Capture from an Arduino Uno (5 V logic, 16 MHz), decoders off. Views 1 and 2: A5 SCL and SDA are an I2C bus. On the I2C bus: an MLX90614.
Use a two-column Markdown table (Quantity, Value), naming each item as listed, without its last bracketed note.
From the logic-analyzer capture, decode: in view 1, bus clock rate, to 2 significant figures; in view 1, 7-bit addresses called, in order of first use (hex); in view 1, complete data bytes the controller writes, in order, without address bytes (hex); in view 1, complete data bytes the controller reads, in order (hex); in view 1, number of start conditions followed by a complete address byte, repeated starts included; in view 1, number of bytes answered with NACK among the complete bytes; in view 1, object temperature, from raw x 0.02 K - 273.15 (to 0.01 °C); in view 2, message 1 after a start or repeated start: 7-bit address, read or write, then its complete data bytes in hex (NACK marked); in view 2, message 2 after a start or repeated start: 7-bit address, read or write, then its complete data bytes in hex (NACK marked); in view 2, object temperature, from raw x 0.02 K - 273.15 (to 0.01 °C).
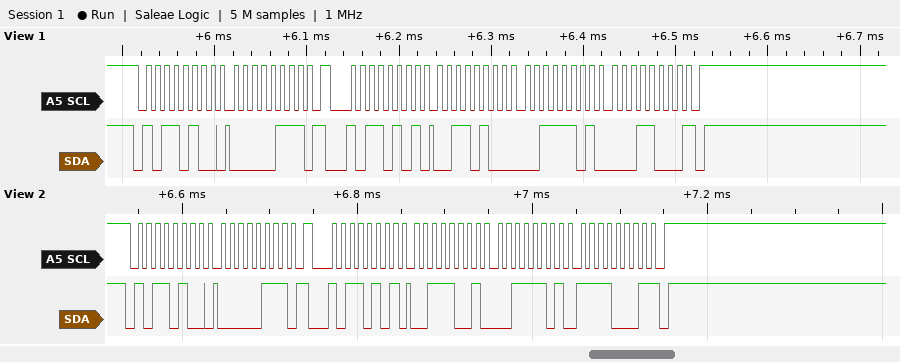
| Quantity | Value |
|---|---|
| in view 1, bus clock rate, to 2 significant figures | 100 kHz |
| in view 1, 7-bit addresses called, in order of first use | 0x5A |
| in view 1, complete data bytes the controller writes, in order, without address bytes | 07 |
| in view 1, complete data bytes the controller reads, in order | 34 3D 18 |
| in view 1, number of start conditions followed by a complete address byte, repeated starts included | 2 |
| in view 1, number of bytes answered with NACK among the complete bytes | 1 |
| in view 1, object temperature, from raw x 0.02 K - 273.15 | 40.21 °C |
| in view 2, message 1 after a start or repeated start: 7-bit address, read or write, then its complete data bytes in hex | 0x5A write: 07 |
| in view 2, message 2 after a start or repeated start: 7-bit address, read or write, then its complete data bytes in hex | 0x5A read: 39 3D F1 NACK |
| in view 2, object temperature, from raw x 0.02 K - 273.15 | 40.31 °C |
